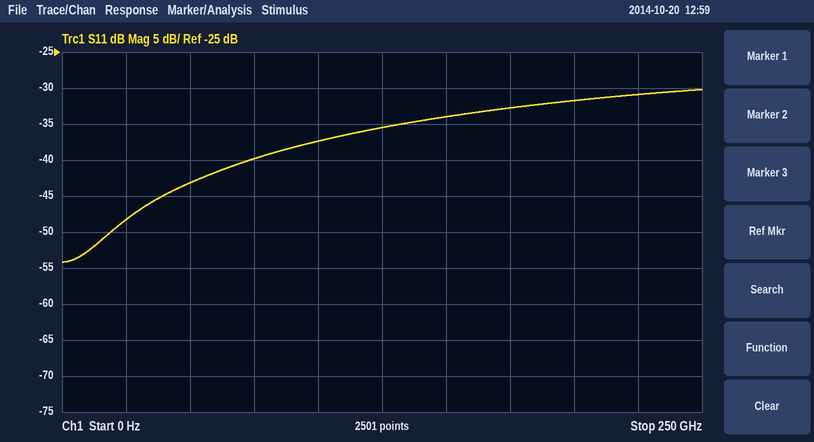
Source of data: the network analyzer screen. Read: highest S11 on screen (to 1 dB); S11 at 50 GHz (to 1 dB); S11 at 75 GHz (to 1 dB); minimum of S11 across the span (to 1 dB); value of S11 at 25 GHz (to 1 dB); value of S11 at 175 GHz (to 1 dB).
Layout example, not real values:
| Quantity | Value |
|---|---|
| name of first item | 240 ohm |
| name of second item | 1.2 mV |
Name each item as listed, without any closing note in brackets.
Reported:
| Quantity | Value |
|---|---|
| highest S11 on screen | -30 dB |
| S11 at 50 GHz | -43 dB |
| S11 at 75 GHz | -40 dB |
| minimum of S11 across the span | -54 dB |
| value of S11 at 25 GHz | -48 dB |
| value of S11 at 175 GHz | -33 dB |
